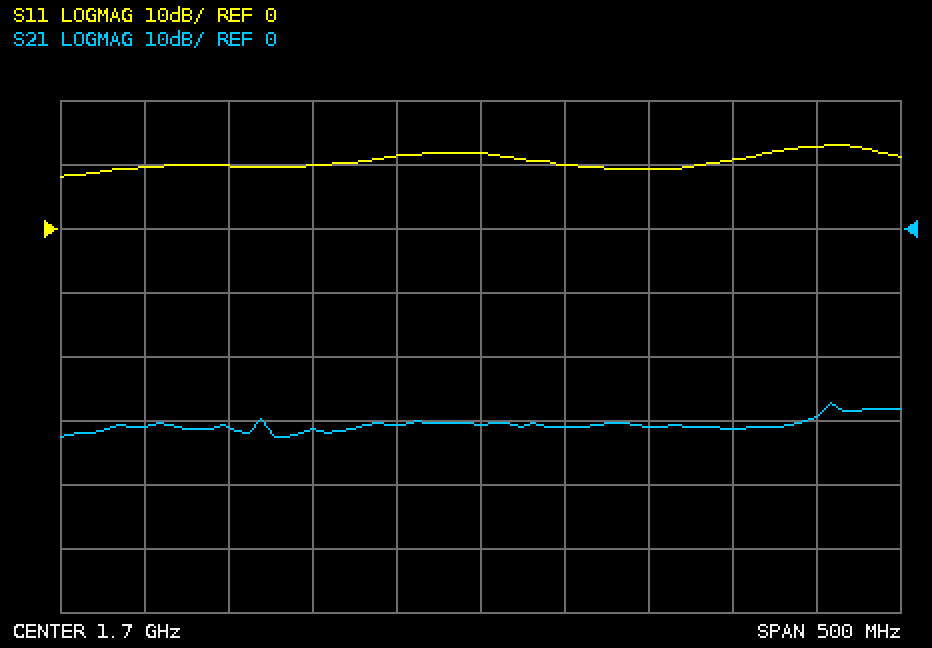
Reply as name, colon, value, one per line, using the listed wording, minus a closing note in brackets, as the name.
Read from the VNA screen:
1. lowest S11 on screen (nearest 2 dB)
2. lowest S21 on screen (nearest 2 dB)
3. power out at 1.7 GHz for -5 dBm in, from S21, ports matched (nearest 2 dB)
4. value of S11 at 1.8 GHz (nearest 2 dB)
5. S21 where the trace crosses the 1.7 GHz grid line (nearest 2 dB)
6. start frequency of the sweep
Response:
lowest S11 on screen: 8 dB
lowest S21 on screen: -32 dB
power out at 1.7 GHz for -5 dBm in, from S21, ports matched: -36 dBm
value of S11 at 1.8 GHz: 10 dB
S21 where the trace crosses the 1.7 GHz grid line: -30 dB
start frequency of the sweep: 1.45 GHz
